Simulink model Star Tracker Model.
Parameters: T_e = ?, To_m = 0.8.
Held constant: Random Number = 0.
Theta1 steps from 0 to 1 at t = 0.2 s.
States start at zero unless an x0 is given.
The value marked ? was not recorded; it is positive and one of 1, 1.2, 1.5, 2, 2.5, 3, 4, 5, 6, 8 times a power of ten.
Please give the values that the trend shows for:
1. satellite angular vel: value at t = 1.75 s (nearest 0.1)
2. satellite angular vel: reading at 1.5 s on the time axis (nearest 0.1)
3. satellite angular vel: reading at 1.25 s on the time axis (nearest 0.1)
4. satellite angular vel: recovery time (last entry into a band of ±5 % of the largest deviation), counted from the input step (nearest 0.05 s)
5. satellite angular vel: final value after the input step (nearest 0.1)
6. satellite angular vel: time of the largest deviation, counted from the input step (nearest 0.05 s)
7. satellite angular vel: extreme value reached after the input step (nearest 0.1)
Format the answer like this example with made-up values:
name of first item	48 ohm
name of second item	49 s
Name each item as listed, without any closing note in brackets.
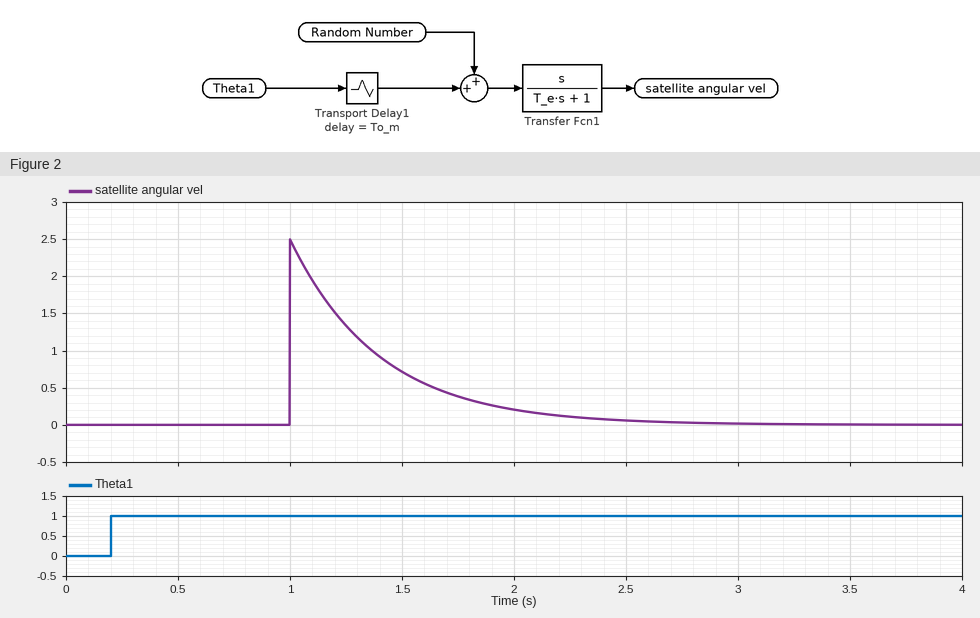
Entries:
satellite angular vel: value at t = 1.75 s	0.4
satellite angular vel: reading at 1.5 s on the time axis	0.7
satellite angular vel: reading at 1.25 s on the time axis	1.3
satellite angular vel: recovery time (last entry into a band of ±5 % of the largest deviation), counted from the input step	2.00 s
satellite angular vel: final value after the input step	0.0
satellite angular vel: time of the largest deviation, counted from the input step	0.80 s
satellite angular vel: extreme value reached after the input step	2.5
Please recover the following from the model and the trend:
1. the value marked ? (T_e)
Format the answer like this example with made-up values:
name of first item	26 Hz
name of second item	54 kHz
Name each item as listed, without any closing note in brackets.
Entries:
the value marked ?	0.4
